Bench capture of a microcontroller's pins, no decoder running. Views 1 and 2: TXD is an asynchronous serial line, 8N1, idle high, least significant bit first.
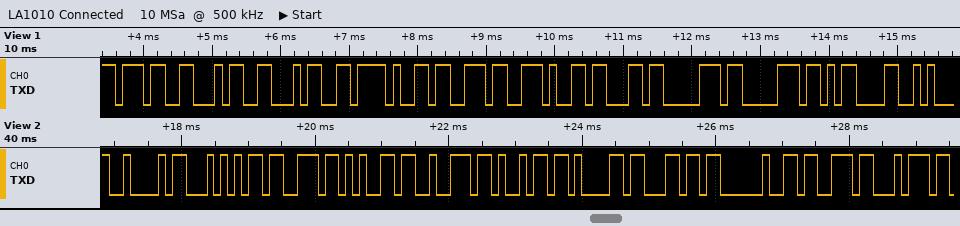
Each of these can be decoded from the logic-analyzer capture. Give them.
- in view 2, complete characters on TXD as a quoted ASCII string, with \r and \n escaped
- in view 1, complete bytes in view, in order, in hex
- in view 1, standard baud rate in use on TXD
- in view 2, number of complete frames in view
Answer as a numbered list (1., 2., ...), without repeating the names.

1. "BTserial st"
2. 37 34 34 2F 73 2E 63 70 70 0D
3. 9600 baud
4. 11
